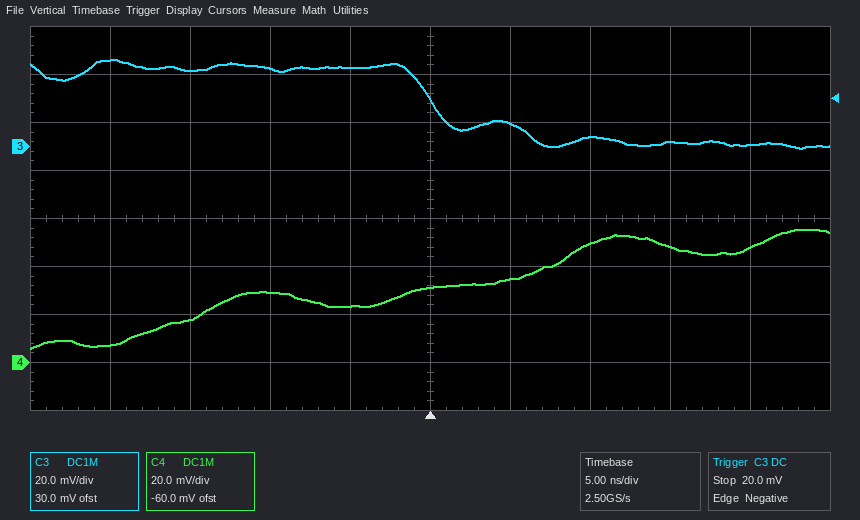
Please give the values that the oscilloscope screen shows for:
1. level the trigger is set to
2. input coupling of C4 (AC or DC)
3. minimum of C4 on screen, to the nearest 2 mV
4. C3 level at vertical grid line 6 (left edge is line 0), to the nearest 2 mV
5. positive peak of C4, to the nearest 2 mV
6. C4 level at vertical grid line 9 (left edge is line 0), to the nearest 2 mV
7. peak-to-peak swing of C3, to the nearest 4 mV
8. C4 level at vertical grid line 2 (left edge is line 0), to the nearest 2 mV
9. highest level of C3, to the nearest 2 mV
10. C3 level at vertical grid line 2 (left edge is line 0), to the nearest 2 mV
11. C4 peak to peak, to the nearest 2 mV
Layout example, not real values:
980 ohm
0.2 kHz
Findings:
20.0 mV
DC
6 mV
10 mV
56 mV
48 mV
36 mV
18 mV
36 mV
32 mV
50 mV
